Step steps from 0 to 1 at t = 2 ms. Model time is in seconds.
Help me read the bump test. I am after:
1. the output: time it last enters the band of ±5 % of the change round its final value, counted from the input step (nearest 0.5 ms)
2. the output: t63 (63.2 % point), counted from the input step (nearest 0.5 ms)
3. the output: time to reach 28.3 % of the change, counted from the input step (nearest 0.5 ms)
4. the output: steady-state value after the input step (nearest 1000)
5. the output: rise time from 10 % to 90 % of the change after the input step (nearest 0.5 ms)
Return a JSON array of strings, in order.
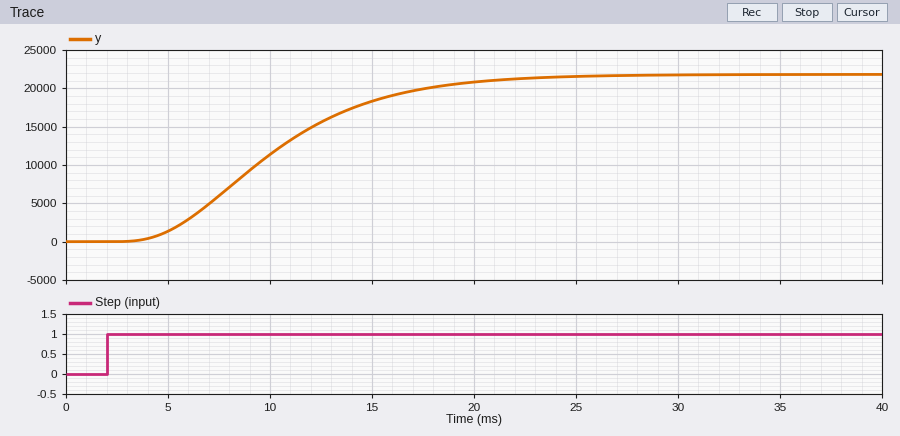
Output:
["17.5 ms", "9.5 ms", "5.5 ms", "22000", "11.5 ms"]
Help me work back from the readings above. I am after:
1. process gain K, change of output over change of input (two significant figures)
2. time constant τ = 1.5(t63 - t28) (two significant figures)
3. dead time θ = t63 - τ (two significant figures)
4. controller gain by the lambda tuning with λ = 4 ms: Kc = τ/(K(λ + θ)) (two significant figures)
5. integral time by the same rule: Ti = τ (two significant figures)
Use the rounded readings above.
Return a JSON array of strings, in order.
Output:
["22000", "6.0 ms", "3.5 ms", "0.000036", "6.0 ms"]
